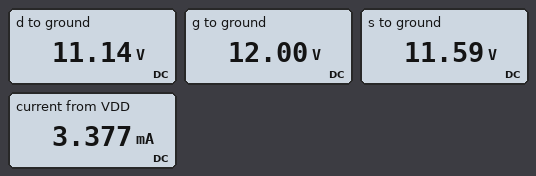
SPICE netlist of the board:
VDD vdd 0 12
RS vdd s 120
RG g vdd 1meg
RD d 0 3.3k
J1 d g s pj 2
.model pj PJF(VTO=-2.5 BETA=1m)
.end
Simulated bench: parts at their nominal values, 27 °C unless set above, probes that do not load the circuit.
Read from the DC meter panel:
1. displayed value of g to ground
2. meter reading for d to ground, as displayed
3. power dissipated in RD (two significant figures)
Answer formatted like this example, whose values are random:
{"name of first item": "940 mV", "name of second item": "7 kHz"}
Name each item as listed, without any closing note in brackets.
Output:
{"displayed value of g to ground": "12.00 V", "meter reading for d to ground, as displayed": "11.14 V", "power dissipated in RD": "38 mW"}
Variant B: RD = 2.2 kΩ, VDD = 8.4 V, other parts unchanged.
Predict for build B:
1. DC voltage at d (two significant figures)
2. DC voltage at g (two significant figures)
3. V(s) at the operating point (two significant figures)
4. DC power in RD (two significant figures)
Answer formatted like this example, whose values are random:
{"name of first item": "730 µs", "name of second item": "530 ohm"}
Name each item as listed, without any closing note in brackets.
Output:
{"DC voltage at d": "7.5 V", "DC voltage at g": "8.4 V", "V(s) at the operating point": "8.0 V", "DC power in RD": "26 mW"}
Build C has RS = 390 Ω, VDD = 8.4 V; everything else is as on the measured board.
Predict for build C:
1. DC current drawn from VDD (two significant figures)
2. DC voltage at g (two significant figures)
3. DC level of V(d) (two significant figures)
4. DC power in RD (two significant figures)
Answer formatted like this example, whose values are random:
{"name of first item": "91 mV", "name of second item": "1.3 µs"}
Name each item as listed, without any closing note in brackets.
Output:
{"DC current drawn from VDD": "2.2 mA", "DC voltage at g": "8.4 V", "DC level of V(d)": "7.2 V", "DC power in RD": "16 mW"}
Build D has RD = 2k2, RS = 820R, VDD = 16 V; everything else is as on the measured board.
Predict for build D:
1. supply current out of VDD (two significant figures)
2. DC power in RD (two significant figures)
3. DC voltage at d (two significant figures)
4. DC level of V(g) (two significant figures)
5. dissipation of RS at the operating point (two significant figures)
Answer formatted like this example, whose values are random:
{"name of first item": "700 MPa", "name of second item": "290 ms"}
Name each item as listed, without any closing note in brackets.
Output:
{"supply current out of VDD": "1.9 mA", "DC power in RD": "7.7 mW", "DC voltage at d": "4.1 V", "DC level of V(g)": "16 V", "dissipation of RS at the operating point": "2.9 mW"}
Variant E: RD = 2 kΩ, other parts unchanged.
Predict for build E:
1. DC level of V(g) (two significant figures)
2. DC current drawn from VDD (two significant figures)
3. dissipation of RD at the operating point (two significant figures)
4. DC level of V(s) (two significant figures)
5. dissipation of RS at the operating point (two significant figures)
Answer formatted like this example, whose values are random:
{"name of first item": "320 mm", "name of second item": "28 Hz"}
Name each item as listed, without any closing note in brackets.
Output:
{"DC level of V(g)": "12 V", "DC current drawn from VDD": "5.2 mA", "dissipation of RD at the operating point": "55 mW", "DC level of V(s)": "11 V", "dissipation of RS at the operating point": "3.3 mW"}
